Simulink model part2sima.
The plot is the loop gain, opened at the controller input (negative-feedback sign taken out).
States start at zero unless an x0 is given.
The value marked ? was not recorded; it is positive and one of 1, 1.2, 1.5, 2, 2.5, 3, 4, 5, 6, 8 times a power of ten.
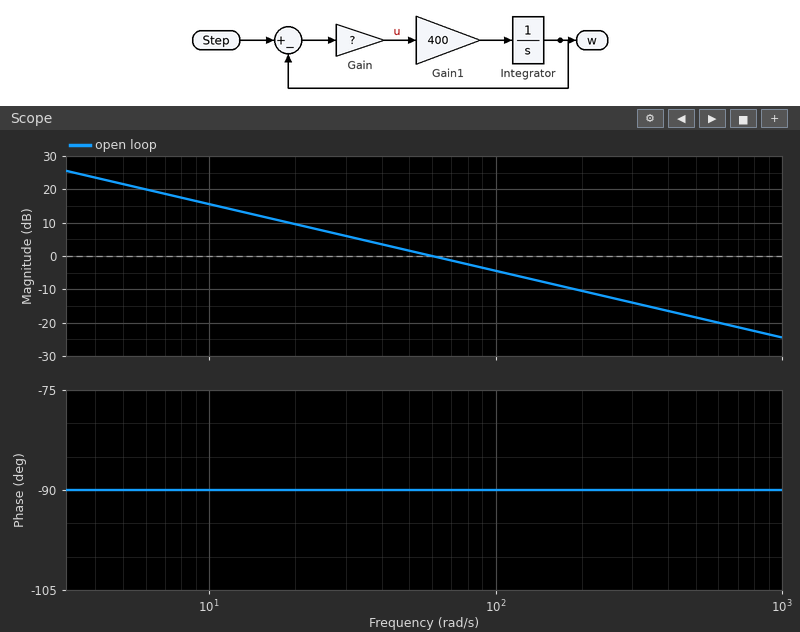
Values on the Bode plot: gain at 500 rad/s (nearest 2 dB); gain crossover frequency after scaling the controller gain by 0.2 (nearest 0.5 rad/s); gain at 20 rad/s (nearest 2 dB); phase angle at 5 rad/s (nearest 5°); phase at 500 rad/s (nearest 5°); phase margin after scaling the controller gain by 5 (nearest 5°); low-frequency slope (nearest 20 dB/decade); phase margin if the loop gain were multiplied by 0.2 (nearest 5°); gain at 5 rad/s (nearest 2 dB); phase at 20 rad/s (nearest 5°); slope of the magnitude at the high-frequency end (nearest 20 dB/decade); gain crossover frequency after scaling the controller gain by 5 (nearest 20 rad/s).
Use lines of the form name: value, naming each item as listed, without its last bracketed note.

gain at 500 rad/s: -18 dB
gain crossover frequency after scaling the controller gain by 0.2: 12.0 rad/s
gain at 20 rad/s: 10 dB
phase angle at 5 rad/s: -90°
phase at 500 rad/s: -90°
phase margin after scaling the controller gain by 5: 90°
low-frequency slope: -20 dB/decade
phase margin if the loop gain were multiplied by 0.2: 90°
gain at 5 rad/s: 22 dB
phase at 20 rad/s: -90°
slope of the magnitude at the high-frequency end: -20 dB/decade
gain crossover frequency after scaling the controller gain by 5: 300 rad/s
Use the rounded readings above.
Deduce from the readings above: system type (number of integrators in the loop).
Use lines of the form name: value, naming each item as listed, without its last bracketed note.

system type: 1
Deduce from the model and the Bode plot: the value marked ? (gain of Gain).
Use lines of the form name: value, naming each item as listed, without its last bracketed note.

the value marked ?: 0.15
